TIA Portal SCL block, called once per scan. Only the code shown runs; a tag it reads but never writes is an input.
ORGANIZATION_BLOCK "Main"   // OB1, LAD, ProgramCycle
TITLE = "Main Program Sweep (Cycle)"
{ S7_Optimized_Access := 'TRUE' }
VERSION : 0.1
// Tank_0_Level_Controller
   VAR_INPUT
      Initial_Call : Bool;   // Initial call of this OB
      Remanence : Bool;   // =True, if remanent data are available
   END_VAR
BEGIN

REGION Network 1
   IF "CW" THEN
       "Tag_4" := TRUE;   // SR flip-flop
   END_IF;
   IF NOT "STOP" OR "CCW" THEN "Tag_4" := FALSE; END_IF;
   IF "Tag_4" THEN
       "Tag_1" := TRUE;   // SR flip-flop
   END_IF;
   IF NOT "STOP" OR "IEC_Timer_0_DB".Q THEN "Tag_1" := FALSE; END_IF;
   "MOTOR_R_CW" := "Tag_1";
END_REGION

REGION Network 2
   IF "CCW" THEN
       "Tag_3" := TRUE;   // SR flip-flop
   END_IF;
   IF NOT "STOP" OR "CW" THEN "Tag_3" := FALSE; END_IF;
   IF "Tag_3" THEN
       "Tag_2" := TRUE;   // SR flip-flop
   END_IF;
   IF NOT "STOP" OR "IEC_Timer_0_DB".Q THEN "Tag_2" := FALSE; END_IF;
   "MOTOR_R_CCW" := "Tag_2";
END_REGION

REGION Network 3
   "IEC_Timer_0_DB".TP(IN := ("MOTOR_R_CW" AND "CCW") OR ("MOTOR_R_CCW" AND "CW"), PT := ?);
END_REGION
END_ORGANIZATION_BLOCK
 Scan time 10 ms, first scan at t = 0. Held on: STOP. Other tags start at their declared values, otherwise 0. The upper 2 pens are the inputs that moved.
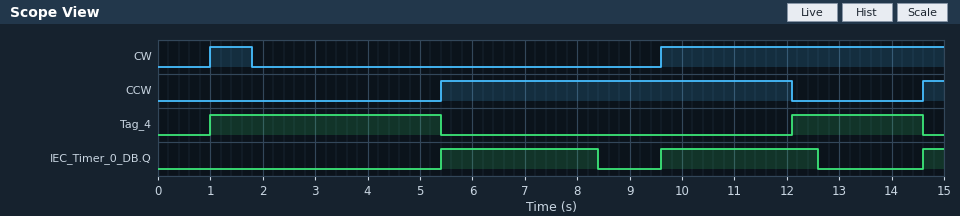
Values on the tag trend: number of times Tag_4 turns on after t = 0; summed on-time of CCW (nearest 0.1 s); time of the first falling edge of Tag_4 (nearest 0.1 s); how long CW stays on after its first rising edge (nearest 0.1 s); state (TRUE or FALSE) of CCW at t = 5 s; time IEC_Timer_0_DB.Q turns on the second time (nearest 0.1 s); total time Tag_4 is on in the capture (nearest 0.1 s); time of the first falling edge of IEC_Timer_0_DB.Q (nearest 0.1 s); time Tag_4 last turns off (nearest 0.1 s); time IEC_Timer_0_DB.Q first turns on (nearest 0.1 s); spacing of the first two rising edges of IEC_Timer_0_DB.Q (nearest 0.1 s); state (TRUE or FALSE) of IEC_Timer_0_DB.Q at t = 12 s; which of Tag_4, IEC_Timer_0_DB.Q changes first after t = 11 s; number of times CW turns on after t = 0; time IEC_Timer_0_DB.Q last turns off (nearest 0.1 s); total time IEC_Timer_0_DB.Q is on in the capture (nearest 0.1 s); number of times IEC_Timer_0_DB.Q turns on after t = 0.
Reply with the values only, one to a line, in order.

2
7.1 s
5.4 s
0.8 s
FALSE
9.6 s
6.9 s
8.4 s
14.6 s
5.4 s
4.2 s
TRUE
Tag_4
2
12.6 s
6.4 s
3
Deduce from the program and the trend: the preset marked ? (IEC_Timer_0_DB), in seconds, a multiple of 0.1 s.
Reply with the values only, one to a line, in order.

3.0 s
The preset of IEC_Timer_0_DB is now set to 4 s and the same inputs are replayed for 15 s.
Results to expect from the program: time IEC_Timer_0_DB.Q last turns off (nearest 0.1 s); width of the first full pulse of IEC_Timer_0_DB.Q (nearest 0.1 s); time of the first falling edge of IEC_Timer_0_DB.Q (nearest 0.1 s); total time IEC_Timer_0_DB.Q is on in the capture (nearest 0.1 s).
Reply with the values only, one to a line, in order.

13.6 s
4.0 s
9.4 s
8.4 s
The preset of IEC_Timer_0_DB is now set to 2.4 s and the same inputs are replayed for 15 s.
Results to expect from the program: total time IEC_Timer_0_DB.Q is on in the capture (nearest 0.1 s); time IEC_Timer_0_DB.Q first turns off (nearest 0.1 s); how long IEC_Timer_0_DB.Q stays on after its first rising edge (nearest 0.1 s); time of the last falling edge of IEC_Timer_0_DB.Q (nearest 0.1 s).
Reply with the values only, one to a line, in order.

5.2 s
7.8 s
2.4 s
12.0 s
